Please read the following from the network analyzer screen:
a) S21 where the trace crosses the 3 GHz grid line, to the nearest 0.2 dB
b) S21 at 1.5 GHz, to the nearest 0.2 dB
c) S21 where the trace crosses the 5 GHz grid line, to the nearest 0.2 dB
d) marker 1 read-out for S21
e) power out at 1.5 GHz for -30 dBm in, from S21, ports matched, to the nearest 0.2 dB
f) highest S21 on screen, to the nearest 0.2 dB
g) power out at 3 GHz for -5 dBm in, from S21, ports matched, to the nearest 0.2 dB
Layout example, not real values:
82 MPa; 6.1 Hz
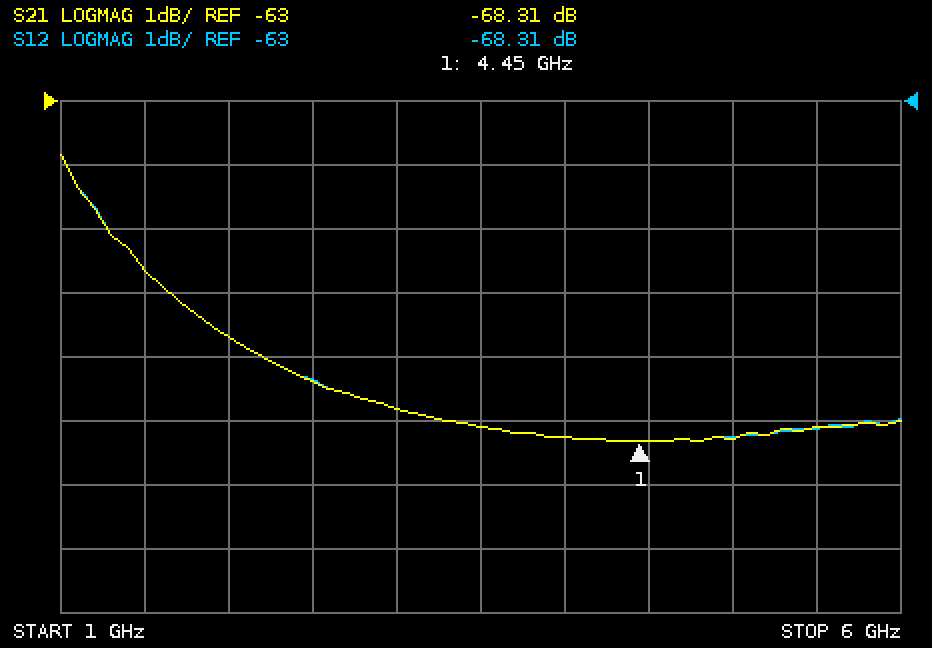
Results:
-67.8 dB; -65.6 dB; -68.2 dB; -68.31 dB; -95.6 dBm; -63.8 dB; -72.8 dBm
